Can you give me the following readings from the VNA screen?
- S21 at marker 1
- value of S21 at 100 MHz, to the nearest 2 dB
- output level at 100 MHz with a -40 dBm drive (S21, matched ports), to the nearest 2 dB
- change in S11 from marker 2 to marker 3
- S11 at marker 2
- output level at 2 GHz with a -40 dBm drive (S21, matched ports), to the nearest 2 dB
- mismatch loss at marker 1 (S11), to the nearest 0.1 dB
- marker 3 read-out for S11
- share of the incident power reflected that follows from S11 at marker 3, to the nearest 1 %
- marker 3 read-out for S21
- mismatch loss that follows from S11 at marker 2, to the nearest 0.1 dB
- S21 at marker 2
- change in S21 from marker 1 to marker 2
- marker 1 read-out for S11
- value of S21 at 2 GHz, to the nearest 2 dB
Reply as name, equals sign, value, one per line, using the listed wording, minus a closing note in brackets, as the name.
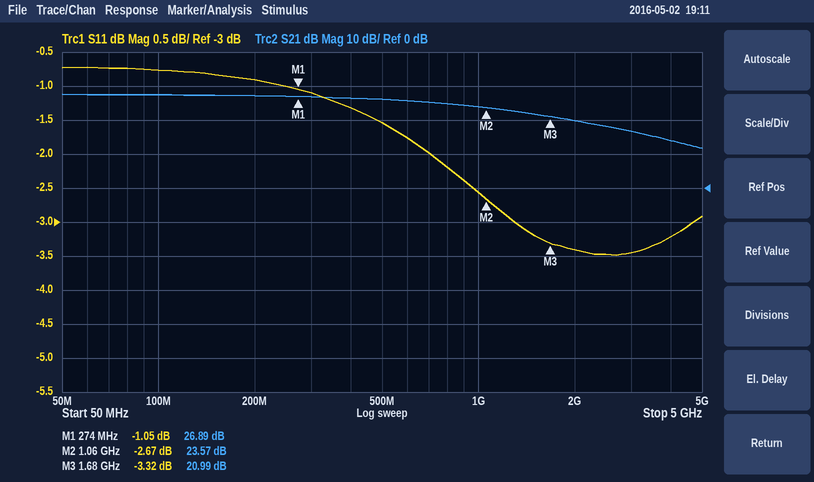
S21 at marker 1 = 26.89 dB
value of S21 at 100 MHz, to the nearest 2 dB = 28 dB
output level at 100 MHz with a -40 dBm drive (S21, matched ports), to the nearest 2 dB = -12 dBm
change in S11 from marker 2 to marker 3 = -0.65 dB
S11 at marker 2 = -2.67 dB
output level at 2 GHz with a -40 dBm drive (S21, matched ports), to the nearest 2 dB = -20 dBm
mismatch loss at marker 1 (S11), to the nearest 0.1 dB = 6.7 dB
marker 3 read-out for S11 = -3.32 dB
share of the incident power reflected that follows from S11 at marker 3, to the nearest 1 % = 47 %
marker 3 read-out for S21 = 20.99 dB
mismatch loss that follows from S11 at marker 2, to the nearest 0.1 dB = 3.4 dB
S21 at marker 2 = 23.57 dB
change in S21 from marker 1 to marker 2 = -3.32 dB
marker 1 read-out for S11 = -1.05 dB
value of S21 at 2 GHz, to the nearest 2 dB = 20 dB
